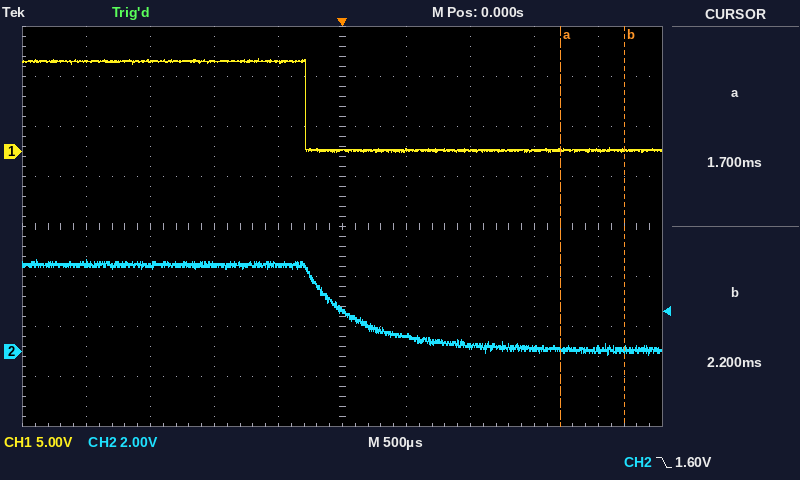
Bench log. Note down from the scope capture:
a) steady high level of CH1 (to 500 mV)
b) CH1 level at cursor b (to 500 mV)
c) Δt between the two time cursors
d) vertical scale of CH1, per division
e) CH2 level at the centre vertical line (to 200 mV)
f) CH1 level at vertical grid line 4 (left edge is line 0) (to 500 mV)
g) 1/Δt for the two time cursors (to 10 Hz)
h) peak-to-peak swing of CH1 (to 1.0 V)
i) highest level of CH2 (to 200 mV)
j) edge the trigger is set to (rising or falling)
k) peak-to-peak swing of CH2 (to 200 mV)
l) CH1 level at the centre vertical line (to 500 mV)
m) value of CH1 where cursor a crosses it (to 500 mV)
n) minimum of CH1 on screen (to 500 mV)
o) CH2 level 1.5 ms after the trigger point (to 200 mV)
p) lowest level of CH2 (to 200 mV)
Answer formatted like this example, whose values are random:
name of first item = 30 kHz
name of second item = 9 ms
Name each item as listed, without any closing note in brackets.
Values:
steady high level of CH1 = 9.0 V
CH1 level at cursor b = 0.0 V
Δt between the two time cursors = 500 µs
vertical scale of CH1, per division = 5 V
CH2 level at the centre vertical line = 1.6 V
CH1 level at vertical grid line 4 (left edge is line 0) = 9.0 V
1/Δt for the two time cursors = 2.00 kHz
peak-to-peak swing of CH1 = 9.0 V
highest level of CH2 = 3.6 V
edge the trigger is set to = falling
peak-to-peak swing of CH2 = 3.8 V
CH1 level at the centre vertical line = 0.0 V
value of CH1 where cursor a crosses it = 0.0 V
minimum of CH1 on screen = 0.0 V
CH2 level 1.5 ms after the trigger point = 200 mV
lowest level of CH2 = -200 mV
